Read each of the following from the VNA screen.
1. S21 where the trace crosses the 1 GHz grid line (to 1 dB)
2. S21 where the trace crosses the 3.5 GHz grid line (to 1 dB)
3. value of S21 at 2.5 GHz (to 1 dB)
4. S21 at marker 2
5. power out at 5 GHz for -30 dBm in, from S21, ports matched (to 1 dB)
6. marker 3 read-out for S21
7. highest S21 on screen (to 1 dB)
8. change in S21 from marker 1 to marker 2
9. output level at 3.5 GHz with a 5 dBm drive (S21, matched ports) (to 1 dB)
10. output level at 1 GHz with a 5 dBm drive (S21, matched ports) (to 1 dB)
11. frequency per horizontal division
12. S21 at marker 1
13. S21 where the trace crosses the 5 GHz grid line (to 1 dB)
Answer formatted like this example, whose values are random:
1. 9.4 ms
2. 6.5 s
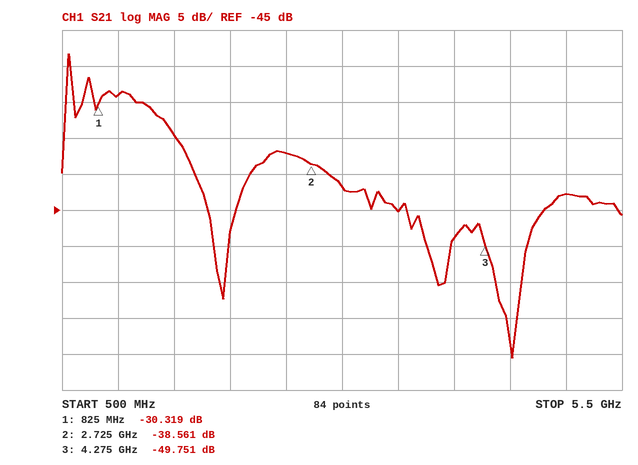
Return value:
1. -29 dB
2. -45 dB
3. -37 dB
4. -38.561 dB
5. -73 dBm
6. -49.751 dB
7. -23 dB
8. -8.242 dB
9. -40 dBm
10. -24 dBm
11. 500 MHz
12. -30.319 dB
13. -43 dB
